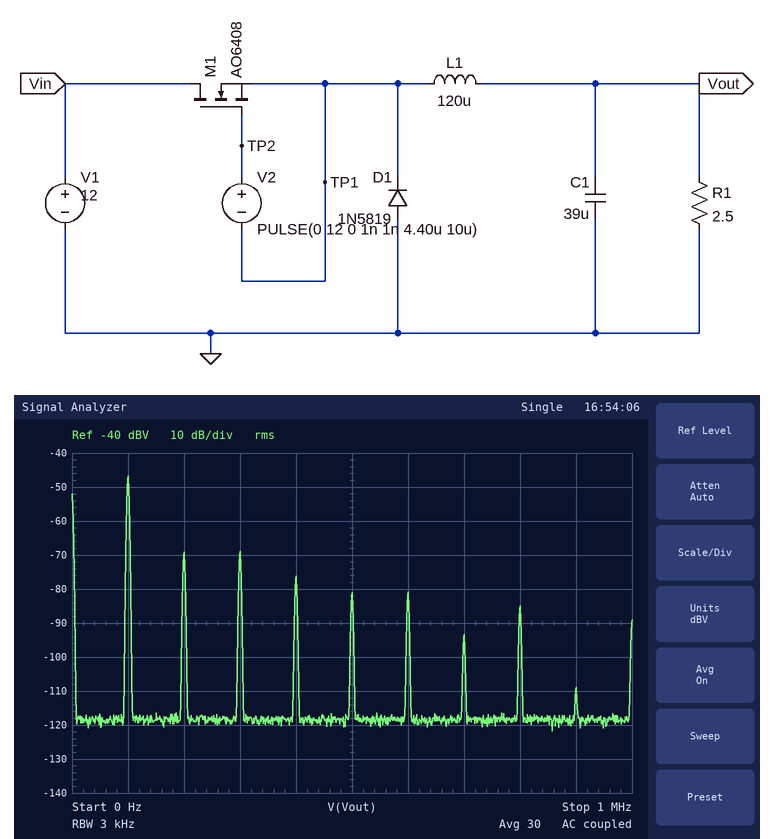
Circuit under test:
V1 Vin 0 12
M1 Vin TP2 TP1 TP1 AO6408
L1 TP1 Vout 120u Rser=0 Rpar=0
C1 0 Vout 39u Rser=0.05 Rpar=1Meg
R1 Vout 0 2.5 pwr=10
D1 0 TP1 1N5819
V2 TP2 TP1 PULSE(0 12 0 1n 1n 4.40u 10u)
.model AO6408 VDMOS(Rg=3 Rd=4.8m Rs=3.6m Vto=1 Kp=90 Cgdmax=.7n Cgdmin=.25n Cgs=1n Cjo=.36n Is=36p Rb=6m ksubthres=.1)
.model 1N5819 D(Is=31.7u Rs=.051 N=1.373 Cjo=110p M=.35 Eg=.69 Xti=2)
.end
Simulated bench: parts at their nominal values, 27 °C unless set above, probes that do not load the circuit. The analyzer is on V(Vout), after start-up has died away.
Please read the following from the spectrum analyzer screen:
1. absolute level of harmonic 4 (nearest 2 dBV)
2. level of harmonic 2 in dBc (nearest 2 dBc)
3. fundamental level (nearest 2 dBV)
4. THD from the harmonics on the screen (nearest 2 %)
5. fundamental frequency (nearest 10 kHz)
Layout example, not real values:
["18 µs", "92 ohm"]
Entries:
["-76 dBV", "-22 dBc", "-46 dBV", "12 %", "100 kHz"]
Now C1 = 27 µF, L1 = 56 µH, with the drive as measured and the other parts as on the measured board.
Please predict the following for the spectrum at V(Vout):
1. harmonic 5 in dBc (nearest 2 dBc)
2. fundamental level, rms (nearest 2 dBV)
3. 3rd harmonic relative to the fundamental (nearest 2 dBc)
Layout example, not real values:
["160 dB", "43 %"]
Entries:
["-36 dBc", "-38 dBV", "-24 dBc"]
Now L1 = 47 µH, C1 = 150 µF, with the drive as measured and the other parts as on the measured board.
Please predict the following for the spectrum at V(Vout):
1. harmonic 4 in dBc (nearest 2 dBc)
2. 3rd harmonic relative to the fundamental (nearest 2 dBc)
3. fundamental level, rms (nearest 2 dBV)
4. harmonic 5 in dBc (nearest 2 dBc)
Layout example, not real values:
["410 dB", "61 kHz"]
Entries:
["-28 dBc", "-20 dBc", "-40 dBV", "-32 dBc"]
